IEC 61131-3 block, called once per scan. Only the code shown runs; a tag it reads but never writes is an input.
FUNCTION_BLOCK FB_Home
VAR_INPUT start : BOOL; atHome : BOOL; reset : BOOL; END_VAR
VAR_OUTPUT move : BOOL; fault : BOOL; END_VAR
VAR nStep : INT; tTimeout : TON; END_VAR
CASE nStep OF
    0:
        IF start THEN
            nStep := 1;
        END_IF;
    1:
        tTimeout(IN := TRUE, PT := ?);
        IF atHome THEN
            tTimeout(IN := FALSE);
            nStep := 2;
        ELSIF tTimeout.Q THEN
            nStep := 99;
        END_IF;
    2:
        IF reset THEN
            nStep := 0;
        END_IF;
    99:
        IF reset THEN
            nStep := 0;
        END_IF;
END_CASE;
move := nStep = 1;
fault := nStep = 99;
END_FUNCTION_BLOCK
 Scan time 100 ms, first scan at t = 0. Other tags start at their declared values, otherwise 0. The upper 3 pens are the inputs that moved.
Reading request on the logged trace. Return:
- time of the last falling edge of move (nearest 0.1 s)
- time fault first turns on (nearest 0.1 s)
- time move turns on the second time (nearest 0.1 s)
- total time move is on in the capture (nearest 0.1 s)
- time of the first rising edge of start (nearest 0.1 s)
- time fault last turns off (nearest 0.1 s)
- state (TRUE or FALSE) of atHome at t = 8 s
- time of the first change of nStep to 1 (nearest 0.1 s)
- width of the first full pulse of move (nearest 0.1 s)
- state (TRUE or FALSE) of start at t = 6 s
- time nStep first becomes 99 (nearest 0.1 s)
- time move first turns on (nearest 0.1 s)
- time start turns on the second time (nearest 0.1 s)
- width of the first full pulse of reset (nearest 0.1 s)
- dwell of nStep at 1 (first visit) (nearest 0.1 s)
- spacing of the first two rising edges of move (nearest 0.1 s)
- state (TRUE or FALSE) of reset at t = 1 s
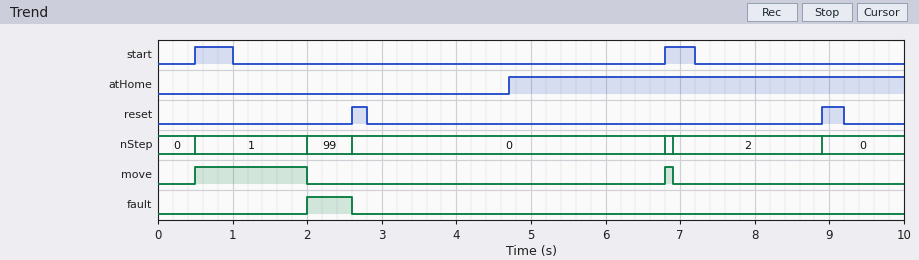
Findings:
6.9 s
2.0 s
6.8 s
1.6 s
0.5 s
2.6 s
TRUE
0.5 s
1.5 s
FALSE
2.0 s
0.5 s
6.8 s
0.2 s
1.5 s
6.3 s
FALSE
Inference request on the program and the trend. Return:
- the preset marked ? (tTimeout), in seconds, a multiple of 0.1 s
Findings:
1.4 s
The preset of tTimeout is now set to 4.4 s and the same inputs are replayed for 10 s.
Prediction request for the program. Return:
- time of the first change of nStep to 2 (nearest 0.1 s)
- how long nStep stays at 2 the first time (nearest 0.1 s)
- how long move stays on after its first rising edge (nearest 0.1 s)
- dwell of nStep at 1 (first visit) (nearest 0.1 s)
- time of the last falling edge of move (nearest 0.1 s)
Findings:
4.7 s
4.2 s
4.2 s
4.2 s
4.7 s
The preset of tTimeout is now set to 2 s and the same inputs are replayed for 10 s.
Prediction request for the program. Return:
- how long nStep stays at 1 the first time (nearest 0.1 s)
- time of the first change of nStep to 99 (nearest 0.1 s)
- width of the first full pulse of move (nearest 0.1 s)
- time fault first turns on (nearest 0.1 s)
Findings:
2.1 s
2.6 s
2.1 s
2.6 s
